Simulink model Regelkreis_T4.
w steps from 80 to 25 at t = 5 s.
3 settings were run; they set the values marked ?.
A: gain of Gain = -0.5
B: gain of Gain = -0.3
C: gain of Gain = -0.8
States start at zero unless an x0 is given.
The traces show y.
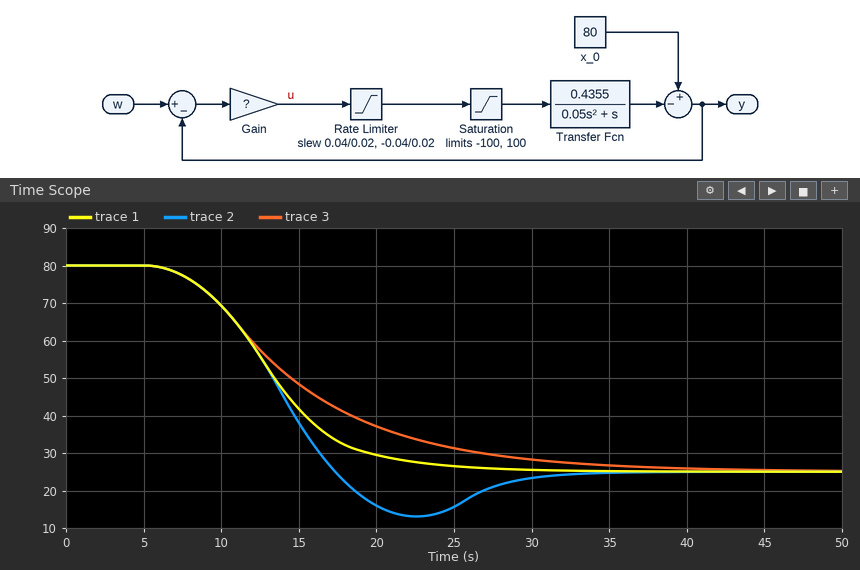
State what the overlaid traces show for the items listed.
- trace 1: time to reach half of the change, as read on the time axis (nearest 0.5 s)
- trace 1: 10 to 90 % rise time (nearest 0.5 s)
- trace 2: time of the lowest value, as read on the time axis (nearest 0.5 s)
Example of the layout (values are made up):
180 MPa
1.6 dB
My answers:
13.0 s
10.5 s
22.5 s
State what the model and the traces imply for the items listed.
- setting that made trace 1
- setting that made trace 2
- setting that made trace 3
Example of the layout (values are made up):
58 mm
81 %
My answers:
A
C
B
